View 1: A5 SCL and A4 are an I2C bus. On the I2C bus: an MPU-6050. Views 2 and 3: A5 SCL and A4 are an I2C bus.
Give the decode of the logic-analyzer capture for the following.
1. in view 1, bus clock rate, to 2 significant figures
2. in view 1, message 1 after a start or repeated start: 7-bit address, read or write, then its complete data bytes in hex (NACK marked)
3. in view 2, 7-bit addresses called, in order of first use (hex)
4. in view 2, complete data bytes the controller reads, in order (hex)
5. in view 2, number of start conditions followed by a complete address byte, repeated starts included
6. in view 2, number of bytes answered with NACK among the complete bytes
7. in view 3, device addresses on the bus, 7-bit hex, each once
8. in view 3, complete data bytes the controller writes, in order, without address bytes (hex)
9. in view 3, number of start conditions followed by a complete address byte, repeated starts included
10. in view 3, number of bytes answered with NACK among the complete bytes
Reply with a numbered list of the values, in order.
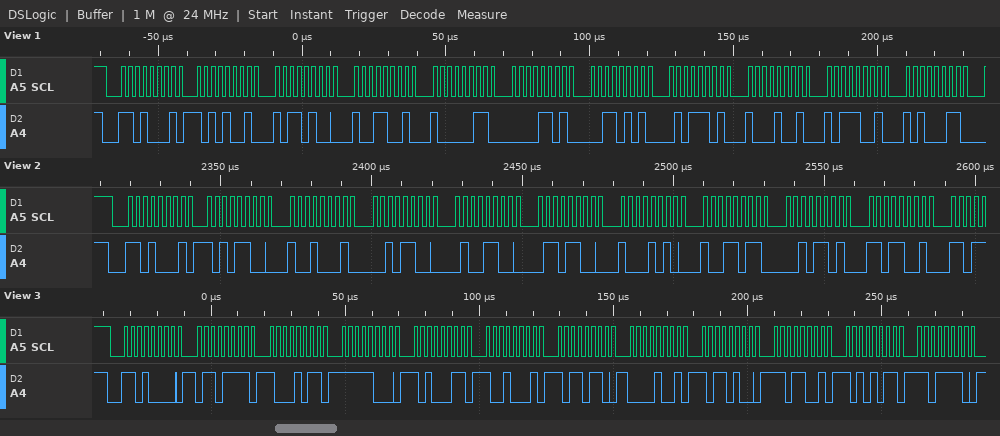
1. 400 kHz
2. 0x68 read: A9 B4 99 83 0D 35 5D 89 B9 A3
3. 0x68
4. AC 91 2C 4C 6C 8A 9B 2D D9
5. 1
6. 0
7. 0x68
8. 6F 8B F8 A3 91 B6 09 B4 D9 AB DE
9. 1
10. 0
